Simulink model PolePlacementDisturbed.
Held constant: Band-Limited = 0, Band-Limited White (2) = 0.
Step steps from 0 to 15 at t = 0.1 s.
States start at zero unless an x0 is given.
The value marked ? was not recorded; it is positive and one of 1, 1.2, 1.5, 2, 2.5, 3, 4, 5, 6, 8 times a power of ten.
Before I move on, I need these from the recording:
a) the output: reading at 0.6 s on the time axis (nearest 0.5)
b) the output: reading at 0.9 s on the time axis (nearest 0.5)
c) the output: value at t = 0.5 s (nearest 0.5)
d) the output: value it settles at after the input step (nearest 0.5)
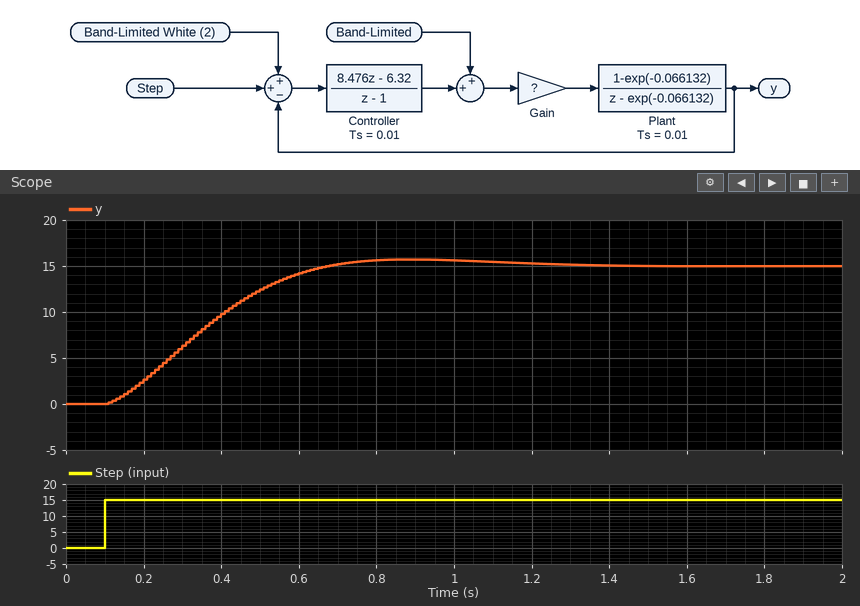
14.0
15.5
12.5
15.0
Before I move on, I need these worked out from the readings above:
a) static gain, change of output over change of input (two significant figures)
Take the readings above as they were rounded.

1.0
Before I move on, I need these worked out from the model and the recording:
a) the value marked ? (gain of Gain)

0.02
